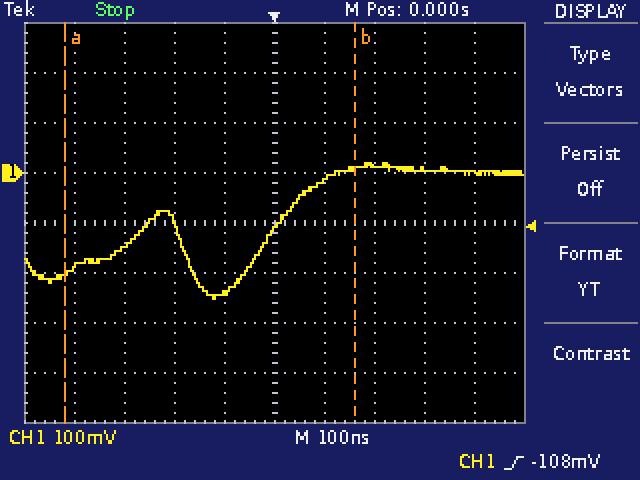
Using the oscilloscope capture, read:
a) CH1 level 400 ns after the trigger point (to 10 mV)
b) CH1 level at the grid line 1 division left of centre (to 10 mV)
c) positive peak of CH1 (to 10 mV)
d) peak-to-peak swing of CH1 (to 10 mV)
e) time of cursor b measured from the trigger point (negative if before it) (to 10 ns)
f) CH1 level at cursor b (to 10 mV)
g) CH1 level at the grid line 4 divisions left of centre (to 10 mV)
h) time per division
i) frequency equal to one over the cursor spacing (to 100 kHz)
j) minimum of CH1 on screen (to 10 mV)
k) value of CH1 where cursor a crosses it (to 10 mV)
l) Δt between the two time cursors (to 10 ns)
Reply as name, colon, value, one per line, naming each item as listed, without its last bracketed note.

CH1 level 400 ns after the trigger point: 0 mV
CH1 level at the grid line 1 division left of centre: -240 mV
positive peak of CH1: 20 mV
peak-to-peak swing of CH1: 270 mV
time of cursor b measured from the trigger point (negative if before it): +160 ns
CH1 level at cursor b: 10 mV
CH1 level at the grid line 4 divisions left of centre: -190 mV
time per division: 100 ns
frequency equal to one over the cursor spacing: 1.7 MHz
minimum of CH1 on screen: -250 mV
value of CH1 where cursor a crosses it: -200 mV
Δt between the two time cursors: 580 ns
